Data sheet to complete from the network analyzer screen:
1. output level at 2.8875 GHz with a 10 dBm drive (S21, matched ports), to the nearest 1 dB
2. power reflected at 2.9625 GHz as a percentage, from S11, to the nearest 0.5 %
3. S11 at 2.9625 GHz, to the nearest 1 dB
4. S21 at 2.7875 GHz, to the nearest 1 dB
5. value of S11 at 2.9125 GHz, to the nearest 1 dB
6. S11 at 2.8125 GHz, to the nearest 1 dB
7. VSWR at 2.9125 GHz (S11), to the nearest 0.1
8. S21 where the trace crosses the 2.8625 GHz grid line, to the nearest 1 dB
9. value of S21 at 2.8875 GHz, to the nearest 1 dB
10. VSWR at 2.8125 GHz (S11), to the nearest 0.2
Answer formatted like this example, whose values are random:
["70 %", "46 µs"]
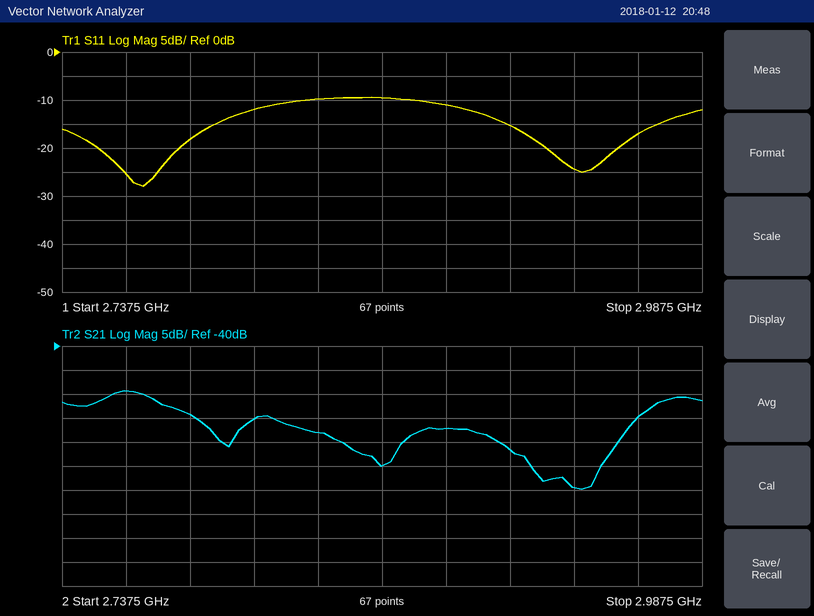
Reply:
["-47 dBm", "2.0 %", "-17 dB", "-54 dB", "-15 dB", "-12 dB", "1.4", "-65 dB", "-57 dB", "1.6"]
